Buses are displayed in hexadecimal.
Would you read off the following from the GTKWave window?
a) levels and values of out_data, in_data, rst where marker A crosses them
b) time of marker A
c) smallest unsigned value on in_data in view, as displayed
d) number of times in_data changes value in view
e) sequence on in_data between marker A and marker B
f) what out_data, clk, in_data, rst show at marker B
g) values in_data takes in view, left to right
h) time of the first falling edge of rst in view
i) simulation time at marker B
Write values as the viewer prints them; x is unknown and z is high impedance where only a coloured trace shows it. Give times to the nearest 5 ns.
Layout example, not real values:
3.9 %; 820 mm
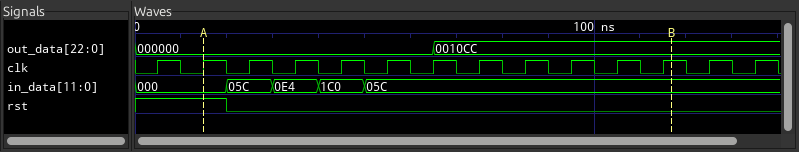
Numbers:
out_data=000000, in_data=000, rst=1; 15 ns; 000; 4; 000, 05C, 0E4, 1C0, 05C; out_data=0010CC, clk=1, in_data=05C, rst=0; 000, 05C, 0E4, 1C0, 05C; 20 ns; 115 ns
